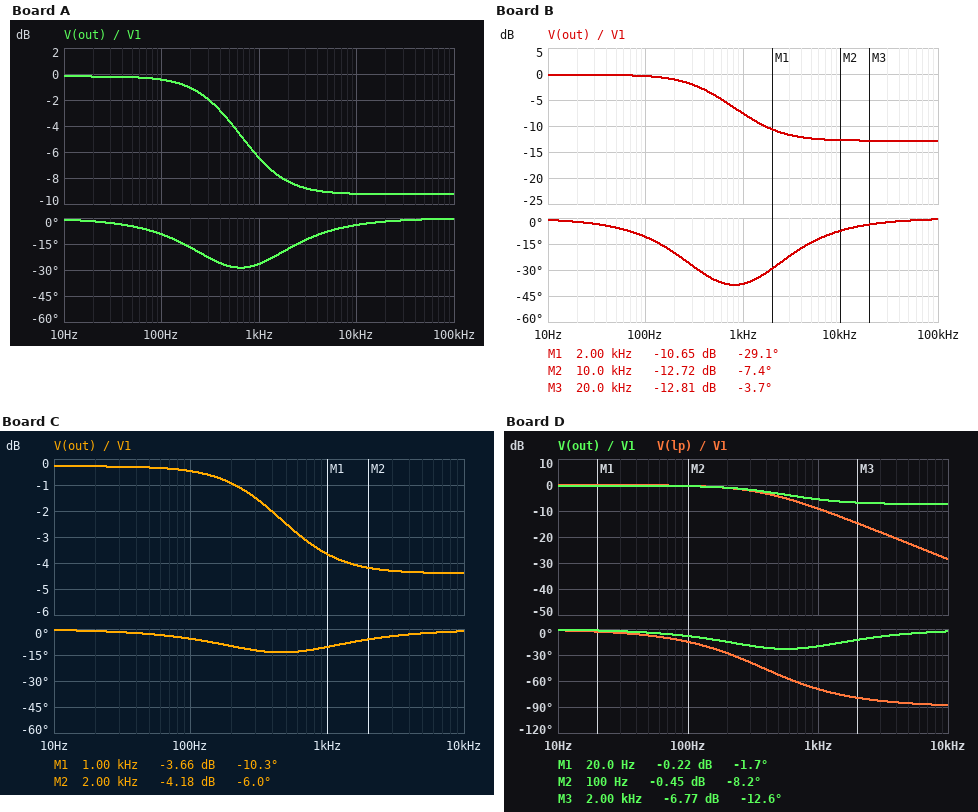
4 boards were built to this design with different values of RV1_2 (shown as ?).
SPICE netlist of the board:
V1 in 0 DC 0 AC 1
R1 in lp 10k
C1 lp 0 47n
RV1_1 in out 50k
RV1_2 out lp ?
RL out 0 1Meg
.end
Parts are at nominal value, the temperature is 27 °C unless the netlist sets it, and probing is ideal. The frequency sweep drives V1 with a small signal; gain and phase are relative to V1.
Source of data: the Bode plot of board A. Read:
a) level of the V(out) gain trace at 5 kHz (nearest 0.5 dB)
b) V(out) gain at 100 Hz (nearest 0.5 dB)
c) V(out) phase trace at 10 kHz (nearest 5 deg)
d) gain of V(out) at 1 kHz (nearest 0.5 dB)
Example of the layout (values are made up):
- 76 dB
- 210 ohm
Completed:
- -9.0 dB
- -0.5 dB
- -5 deg
- -6.5 dB
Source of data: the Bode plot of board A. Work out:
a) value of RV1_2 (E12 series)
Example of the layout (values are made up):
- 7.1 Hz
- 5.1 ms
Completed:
- 27 kΩ
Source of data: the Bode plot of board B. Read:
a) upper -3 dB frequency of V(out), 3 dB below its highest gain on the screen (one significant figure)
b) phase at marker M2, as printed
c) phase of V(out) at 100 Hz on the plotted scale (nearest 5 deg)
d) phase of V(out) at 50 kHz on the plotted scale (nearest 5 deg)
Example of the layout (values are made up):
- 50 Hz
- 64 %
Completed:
- 400 Hz
- -7.4 deg
- -10 deg
- 0 deg
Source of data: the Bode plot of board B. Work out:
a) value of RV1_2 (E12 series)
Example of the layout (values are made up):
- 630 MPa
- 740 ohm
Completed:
- 15 kΩ
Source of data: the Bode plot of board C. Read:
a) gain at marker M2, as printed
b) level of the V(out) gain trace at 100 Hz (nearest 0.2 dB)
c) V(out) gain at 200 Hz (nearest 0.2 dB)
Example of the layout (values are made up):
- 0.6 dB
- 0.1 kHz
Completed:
- -4.18 dB
- -0.4 dB
- -1.0 dB
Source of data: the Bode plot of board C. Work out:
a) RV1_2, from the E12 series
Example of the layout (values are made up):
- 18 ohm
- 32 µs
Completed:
- 82 kΩ
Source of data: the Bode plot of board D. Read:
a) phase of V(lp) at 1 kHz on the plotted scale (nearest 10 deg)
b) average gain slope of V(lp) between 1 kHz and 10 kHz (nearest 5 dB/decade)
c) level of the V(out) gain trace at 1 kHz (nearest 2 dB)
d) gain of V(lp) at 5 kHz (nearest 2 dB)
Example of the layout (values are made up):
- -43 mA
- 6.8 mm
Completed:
- -70 deg
- -20 dB/decade
- -6 dB
- -22 dB
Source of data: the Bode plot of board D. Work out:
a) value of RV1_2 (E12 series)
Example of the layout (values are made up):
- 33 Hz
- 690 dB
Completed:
- 39 kΩ
